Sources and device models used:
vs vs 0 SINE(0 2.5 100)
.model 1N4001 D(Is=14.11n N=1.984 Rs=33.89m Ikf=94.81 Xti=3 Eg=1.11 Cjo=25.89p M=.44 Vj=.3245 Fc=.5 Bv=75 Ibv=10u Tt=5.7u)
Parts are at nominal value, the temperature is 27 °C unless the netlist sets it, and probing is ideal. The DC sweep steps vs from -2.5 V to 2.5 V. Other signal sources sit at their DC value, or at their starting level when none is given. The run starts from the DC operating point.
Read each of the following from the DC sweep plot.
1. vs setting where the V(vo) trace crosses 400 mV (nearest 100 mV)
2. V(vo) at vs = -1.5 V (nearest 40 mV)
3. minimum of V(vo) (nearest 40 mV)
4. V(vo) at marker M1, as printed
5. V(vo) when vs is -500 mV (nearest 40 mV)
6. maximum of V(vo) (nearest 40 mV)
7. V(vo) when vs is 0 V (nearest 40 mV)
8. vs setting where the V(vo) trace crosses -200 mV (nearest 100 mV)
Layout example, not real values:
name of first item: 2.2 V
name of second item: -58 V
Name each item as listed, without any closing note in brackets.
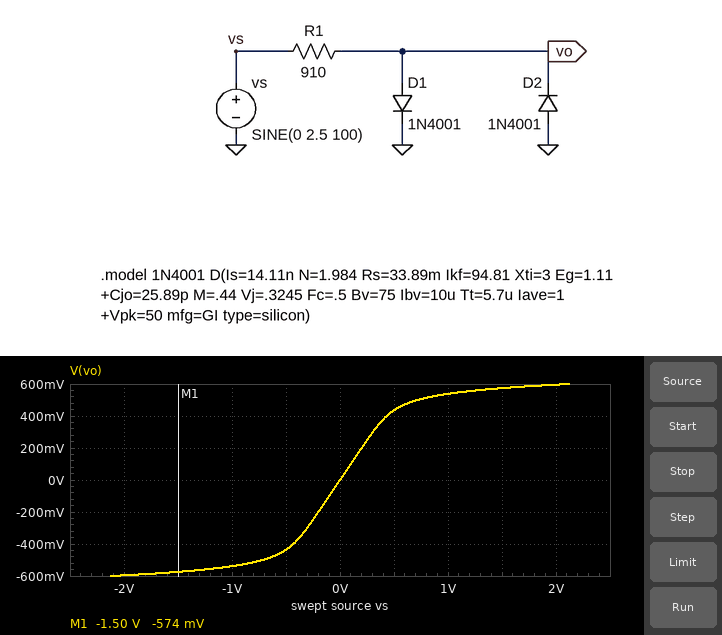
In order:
vs setting where the V(vo) trace crosses 400 mV: 400 mV
V(vo) at vs = -1.5 V: -560 mV
minimum of V(vo): -600 mV
V(vo) at marker M1, as printed: -574 mV
V(vo) when vs is -500 mV: -440 mV
maximum of V(vo): 600 mV
V(vo) when vs is 0 V: 0 V
vs setting where the V(vo) trace crosses -200 mV: -200 mV
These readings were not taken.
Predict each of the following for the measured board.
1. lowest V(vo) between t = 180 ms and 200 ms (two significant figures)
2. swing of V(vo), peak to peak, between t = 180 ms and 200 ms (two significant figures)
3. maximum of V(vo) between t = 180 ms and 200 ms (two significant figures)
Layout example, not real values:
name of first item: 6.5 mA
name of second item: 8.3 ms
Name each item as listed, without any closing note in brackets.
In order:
lowest V(vo) between t = 180 ms and 200 ms: -610 mV
swing of V(vo), peak to peak, between t = 180 ms and 200 ms: 1.2 V
maximum of V(vo) between t = 180 ms and 200 ms: 610 mV
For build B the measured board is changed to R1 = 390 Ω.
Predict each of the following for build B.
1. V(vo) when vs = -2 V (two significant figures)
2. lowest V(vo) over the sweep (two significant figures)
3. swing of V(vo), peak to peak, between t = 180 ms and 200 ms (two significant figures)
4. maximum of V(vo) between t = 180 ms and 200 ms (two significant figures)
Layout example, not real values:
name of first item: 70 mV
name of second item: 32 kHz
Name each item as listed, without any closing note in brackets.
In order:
V(vo) when vs = -2 V: -640 mV
lowest V(vo) over the sweep: -650 mV
swing of V(vo), peak to peak, between t = 180 ms and 200 ms: 1.3 V
maximum of V(vo) between t = 180 ms and 200 ms: 650 mV
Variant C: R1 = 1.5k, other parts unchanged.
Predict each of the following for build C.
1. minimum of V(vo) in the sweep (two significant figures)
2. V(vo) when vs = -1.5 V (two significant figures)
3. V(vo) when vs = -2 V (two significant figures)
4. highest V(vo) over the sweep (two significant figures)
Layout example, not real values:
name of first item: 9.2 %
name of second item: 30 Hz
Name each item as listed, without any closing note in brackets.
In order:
minimum of V(vo) in the sweep: -590 mV
V(vo) when vs = -1.5 V: -550 mV
V(vo) when vs = -2 V: -570 mV
highest V(vo) over the sweep: 590 mV
